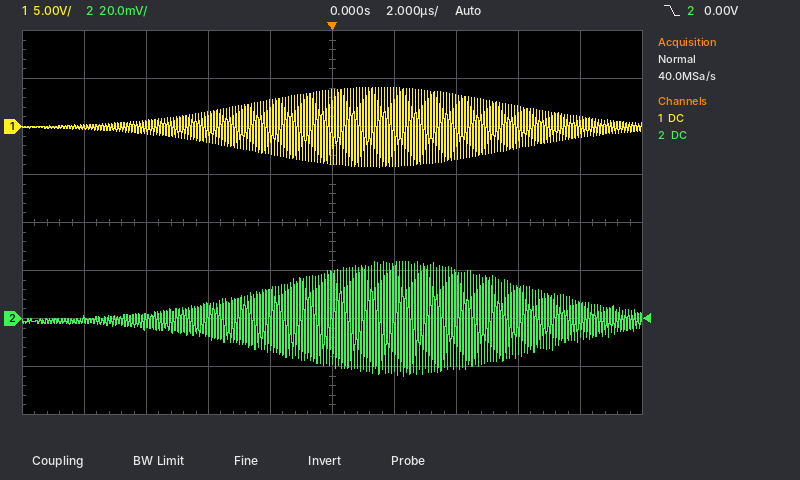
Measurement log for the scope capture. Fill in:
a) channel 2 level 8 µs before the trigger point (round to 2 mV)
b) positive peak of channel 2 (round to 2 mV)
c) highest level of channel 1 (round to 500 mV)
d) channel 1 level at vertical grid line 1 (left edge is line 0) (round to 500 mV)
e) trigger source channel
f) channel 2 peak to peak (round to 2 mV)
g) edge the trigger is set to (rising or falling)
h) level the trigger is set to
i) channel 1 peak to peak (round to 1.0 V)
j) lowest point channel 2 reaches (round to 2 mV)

0 mV
24 mV
4.0 V
0.0 V
channel 2
48 mV
falling
0.00 V
8.0 V
-24 mV
